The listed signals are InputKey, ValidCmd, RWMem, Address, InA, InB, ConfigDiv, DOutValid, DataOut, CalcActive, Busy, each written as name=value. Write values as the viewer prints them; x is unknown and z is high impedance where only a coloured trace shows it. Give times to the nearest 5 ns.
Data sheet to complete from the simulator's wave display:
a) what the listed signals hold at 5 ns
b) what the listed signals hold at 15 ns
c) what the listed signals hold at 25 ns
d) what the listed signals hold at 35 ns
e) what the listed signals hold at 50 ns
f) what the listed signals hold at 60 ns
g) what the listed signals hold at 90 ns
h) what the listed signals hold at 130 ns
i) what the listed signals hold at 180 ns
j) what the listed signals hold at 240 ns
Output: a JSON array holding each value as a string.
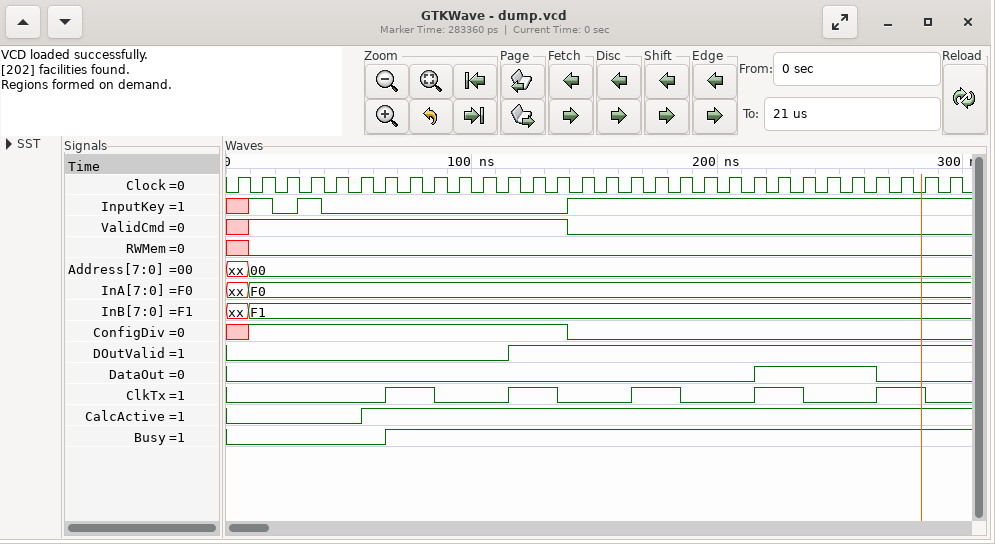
["InputKey=x, ValidCmd=x, RWMem=x, Address=xx, InA=xx, InB=xx, ConfigDiv=x, DOutValid=0, DataOut=0, CalcActive=0, Busy=0", "InputKey=1, ValidCmd=1, RWMem=0, Address=00, InA=F0, InB=F1, ConfigDiv=1, DOutValid=0, DataOut=0, CalcActive=0, Busy=0", "InputKey=0, ValidCmd=1, RWMem=0, Address=00, InA=F0, InB=F1, ConfigDiv=1, DOutValid=0, DataOut=0, CalcActive=0, Busy=0", "InputKey=1, ValidCmd=1, RWMem=0, Address=00, InA=F0, InB=F1, ConfigDiv=1, DOutValid=0, DataOut=0, CalcActive=0, Busy=0", "InputKey=0, ValidCmd=1, RWMem=0, Address=00, InA=F0, InB=F1, ConfigDiv=1, DOutValid=0, DataOut=0, CalcActive=0, Busy=0", "InputKey=0, ValidCmd=1, RWMem=0, Address=00, InA=F0, InB=F1, ConfigDiv=1, DOutValid=0, DataOut=0, CalcActive=1, Busy=0", "InputKey=0, ValidCmd=1, RWMem=0, Address=00, InA=F0, InB=F1, ConfigDiv=1, DOutValid=0, DataOut=0, CalcActive=1, Busy=1", "InputKey=0, ValidCmd=1, RWMem=0, Address=00, InA=F0, InB=F1, ConfigDiv=1, DOutValid=1, DataOut=0, CalcActive=1, Busy=1", "InputKey=1, ValidCmd=0, RWMem=0, Address=00, InA=F0, InB=F1, ConfigDiv=0, DOutValid=1, DataOut=0, CalcActive=1, Busy=1", "InputKey=1, ValidCmd=0, RWMem=0, Address=00, InA=F0, InB=F1, ConfigDiv=0, DOutValid=1, DataOut=1, CalcActive=1, Busy=1"]
